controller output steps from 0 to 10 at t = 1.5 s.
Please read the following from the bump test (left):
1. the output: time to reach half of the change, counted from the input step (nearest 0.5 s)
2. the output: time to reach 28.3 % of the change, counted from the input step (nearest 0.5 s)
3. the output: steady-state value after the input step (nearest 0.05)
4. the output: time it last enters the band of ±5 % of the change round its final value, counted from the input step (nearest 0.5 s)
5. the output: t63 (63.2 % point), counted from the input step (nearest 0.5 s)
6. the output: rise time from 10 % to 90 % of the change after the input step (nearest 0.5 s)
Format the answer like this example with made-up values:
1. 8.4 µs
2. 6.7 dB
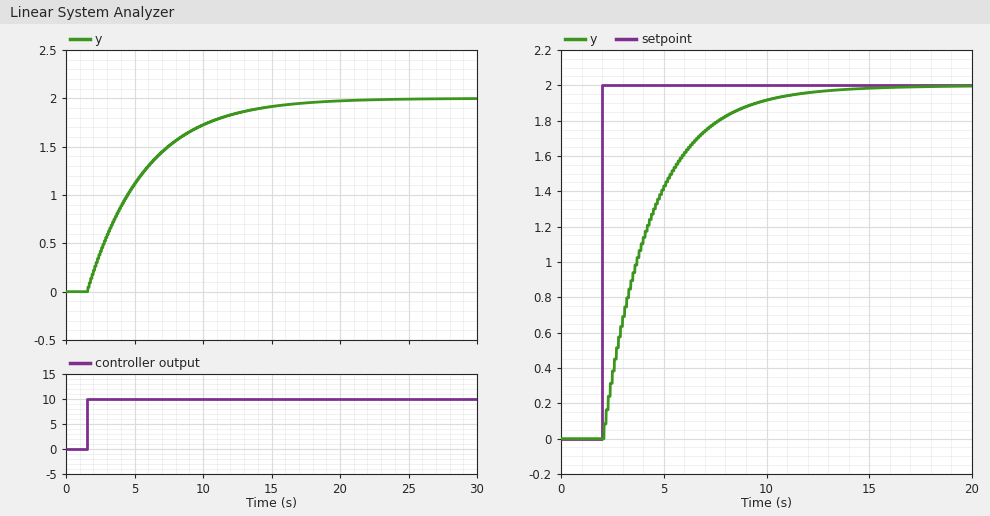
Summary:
1. 3.0 s
2. 1.5 s
3. 2.00
4. 13.0 s
5. 4.5 s
6. 9.5 s
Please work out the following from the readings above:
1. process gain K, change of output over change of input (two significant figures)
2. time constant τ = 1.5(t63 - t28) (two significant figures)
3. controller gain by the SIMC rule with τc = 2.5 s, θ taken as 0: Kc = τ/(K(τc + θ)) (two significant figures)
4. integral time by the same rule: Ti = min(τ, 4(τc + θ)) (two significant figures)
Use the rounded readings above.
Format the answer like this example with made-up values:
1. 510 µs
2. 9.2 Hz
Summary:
1. 0.20
2. 4.5 s
3. 9.0
4. 4.5 s
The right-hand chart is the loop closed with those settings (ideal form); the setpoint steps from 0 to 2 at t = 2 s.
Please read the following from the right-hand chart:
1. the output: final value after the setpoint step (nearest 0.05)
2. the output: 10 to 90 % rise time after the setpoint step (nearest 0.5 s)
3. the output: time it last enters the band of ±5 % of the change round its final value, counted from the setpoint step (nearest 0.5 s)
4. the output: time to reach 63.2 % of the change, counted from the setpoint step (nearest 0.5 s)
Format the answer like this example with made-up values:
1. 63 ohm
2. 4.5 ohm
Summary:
1. 2.00
2. 5.5 s
3. 7.5 s
4. 2.5 s
